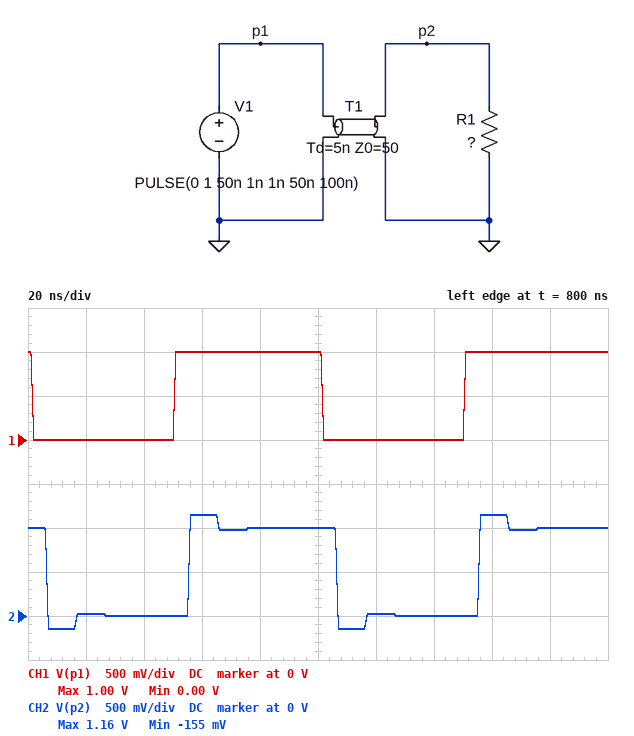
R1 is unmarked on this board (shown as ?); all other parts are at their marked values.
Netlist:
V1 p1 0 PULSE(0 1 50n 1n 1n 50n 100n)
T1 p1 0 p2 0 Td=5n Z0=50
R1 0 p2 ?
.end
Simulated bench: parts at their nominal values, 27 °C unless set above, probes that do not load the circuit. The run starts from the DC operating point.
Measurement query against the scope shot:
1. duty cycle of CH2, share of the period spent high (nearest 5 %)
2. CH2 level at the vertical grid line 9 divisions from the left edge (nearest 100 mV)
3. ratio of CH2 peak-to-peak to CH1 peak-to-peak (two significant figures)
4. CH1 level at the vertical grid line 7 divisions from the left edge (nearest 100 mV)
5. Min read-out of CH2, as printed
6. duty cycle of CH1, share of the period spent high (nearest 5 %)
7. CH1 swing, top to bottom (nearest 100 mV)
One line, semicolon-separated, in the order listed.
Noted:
50 %; 1.0 V; 1.3; 0 V; -155 mV; 50 %; 1.0 V
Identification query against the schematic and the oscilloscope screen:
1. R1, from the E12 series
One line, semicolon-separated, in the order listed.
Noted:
68 Ω
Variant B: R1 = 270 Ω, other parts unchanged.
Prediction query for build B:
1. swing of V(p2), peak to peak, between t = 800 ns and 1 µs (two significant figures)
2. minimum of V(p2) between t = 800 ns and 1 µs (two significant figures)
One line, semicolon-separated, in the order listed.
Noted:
2.6 V; -810 mV
